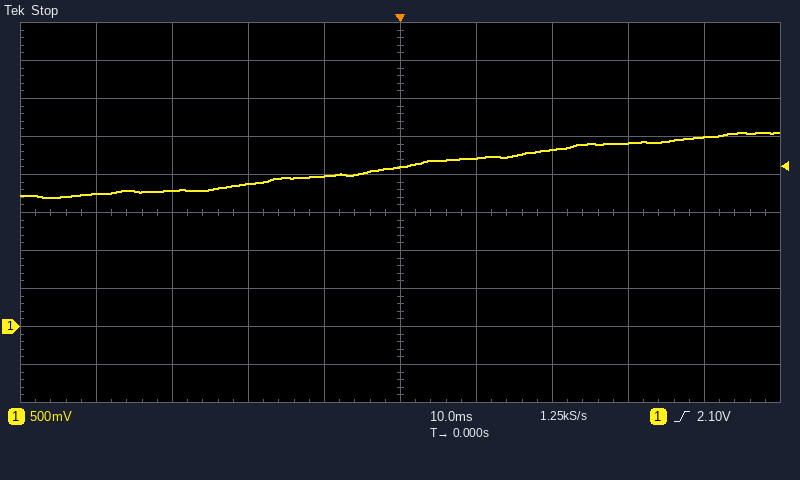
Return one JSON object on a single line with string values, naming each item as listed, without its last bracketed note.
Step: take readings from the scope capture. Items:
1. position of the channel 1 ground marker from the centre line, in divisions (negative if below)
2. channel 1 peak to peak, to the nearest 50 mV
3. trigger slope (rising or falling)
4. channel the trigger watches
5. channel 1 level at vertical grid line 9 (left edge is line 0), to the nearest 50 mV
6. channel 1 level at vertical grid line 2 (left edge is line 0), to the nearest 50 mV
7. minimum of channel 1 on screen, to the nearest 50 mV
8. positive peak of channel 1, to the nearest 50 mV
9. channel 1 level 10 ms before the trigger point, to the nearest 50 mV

{"position of the channel 1 ground marker from the centre line, in divisions": "-3.0 div", "channel 1 peak to peak, to the nearest 50 mV": "850 mV", "trigger slope": "rising", "channel the trigger watches": "channel 1", "channel 1 level at vertical grid line 9 (left edge is line 0), to the nearest 50 mV": "2.50 V", "channel 1 level at vertical grid line 2 (left edge is line 0), to the nearest 50 mV": "1.80 V", "minimum of channel 1 on screen, to the nearest 50 mV": "1.70 V", "positive peak of channel 1, to the nearest 50 mV": "2.55 V", "channel 1 level 10 ms before the trigger point, to the nearest 50 mV": "2.00 V"}
